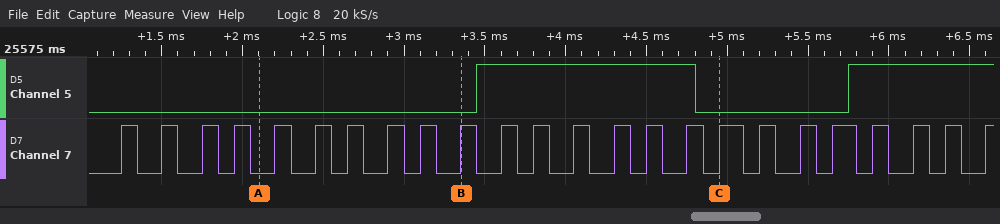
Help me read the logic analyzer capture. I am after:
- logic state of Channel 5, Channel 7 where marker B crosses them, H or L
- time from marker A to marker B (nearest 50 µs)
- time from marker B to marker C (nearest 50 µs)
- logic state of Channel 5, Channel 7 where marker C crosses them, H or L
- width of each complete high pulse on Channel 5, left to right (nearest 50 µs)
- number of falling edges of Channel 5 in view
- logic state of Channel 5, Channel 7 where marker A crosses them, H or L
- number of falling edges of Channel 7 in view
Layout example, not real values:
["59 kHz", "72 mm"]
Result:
["Channel 5=L, Channel 7=H", "1250 µs", "1600 µs", "Channel 5=L, Channel 7=H", "1350 µs", "1", "Channel 5=L, Channel 7=L", "23"]
